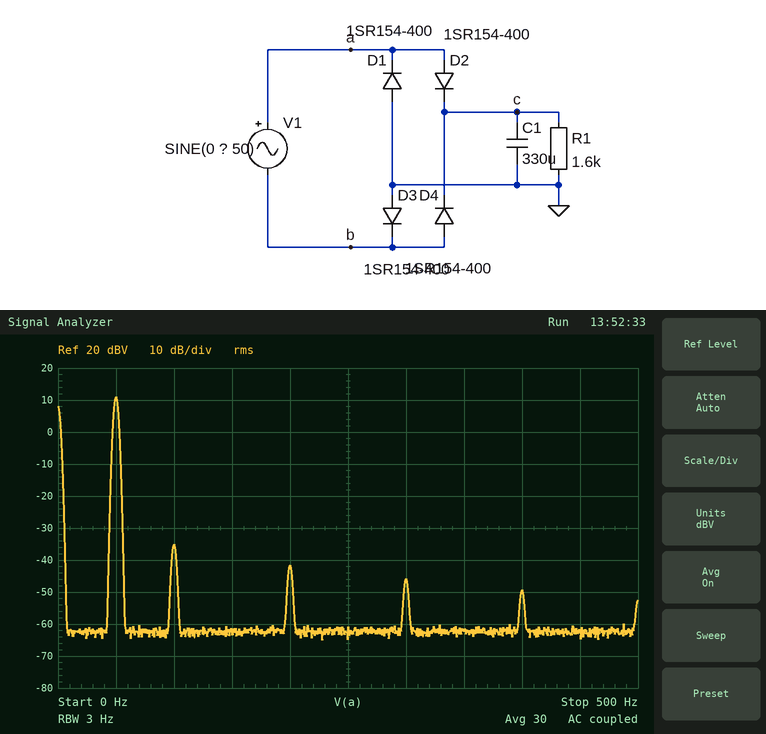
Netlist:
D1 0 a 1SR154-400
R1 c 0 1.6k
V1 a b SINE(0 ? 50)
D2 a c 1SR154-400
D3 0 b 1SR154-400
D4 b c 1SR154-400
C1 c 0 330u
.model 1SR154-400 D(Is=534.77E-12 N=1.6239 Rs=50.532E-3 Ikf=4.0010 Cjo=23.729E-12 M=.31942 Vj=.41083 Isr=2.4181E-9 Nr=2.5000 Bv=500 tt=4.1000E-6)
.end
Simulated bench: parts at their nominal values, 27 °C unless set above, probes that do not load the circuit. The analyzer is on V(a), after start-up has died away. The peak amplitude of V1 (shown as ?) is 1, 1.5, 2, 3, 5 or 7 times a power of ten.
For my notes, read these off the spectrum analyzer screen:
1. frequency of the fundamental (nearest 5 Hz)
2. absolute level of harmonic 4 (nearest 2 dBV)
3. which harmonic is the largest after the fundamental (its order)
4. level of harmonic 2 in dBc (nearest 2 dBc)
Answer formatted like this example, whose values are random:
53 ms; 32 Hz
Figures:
50 Hz; -42 dBV; 2; -46 dBc
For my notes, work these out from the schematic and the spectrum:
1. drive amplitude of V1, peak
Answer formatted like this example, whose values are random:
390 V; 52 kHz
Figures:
10 V
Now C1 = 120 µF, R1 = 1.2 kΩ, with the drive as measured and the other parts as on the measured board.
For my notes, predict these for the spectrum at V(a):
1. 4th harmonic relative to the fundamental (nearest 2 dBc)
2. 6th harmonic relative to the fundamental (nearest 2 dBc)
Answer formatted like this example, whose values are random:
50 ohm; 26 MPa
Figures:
-42 dBc; -46 dBc
